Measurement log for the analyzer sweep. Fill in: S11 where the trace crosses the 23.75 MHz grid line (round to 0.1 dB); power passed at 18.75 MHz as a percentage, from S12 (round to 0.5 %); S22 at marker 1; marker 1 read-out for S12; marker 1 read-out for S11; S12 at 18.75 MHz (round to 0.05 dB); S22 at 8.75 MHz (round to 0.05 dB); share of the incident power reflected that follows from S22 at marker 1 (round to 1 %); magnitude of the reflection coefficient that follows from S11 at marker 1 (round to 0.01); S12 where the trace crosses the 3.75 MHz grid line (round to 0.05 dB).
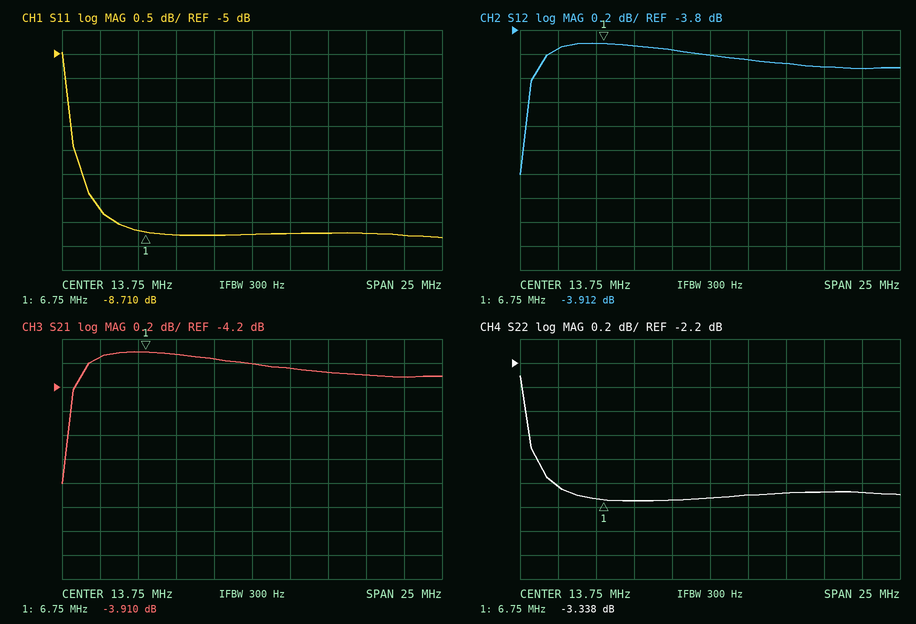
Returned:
-8.8 dB
39.0 %
-3.338 dB
-3.912 dB
-8.710 dB
-4.10 dB
-3.35 dB
46 %
0.37
-3.95 dB
